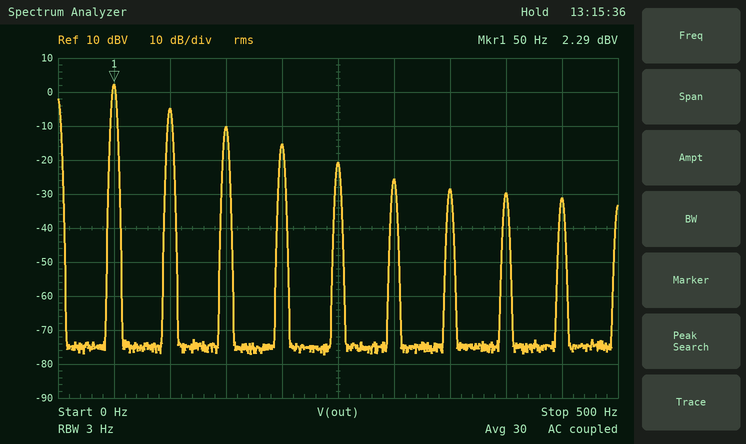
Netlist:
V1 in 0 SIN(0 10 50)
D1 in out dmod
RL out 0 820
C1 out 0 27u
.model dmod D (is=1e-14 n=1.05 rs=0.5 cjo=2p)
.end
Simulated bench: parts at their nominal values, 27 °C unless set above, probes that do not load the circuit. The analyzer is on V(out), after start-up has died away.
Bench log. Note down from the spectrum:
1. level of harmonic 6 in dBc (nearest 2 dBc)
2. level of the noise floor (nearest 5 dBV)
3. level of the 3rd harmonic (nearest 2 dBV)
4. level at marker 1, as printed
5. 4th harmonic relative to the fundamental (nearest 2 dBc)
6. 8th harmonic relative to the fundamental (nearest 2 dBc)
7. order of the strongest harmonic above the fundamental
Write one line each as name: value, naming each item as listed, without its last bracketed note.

level of harmonic 6 in dBc: -28 dBc
level of the noise floor: -75 dBV
level of the 3rd harmonic: -10 dBV
level at marker 1, as printed: 2.29 dBV
4th harmonic relative to the fundamental: -18 dBc
8th harmonic relative to the fundamental: -32 dBc
order of the strongest harmonic above the fundamental: 2
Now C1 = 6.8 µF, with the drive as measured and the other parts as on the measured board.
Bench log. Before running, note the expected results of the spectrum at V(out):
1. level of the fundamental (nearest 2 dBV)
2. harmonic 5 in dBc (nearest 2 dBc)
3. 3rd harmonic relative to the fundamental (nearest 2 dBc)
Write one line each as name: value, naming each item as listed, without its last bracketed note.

level of the fundamental: 8 dBV
harmonic 5 in dBc: -28 dBc
3rd harmonic relative to the fundamental: -18 dBc
